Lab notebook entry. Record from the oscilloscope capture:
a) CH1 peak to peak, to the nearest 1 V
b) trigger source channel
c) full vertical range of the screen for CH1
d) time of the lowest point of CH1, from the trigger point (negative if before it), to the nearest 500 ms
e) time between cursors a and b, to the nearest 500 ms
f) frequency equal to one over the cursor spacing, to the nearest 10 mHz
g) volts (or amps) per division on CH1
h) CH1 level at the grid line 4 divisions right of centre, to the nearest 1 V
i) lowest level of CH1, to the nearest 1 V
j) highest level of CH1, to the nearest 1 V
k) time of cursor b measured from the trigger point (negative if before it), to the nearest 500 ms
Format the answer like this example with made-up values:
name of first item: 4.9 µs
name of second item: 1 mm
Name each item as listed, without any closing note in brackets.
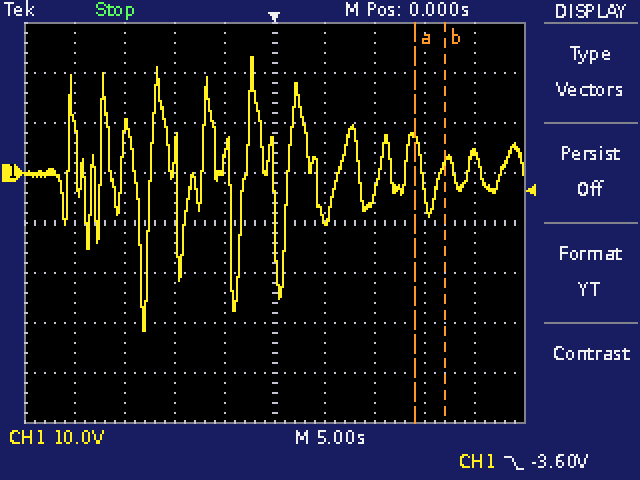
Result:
CH1 peak to peak, to the nearest 1 V: 55 V
trigger source channel: CH1
full vertical range of the screen for CH1: 80 V
time of the lowest point of CH1, from the trigger point (negative if before it), to the nearest 500 ms: -13.0 s
time between cursors a and b, to the nearest 500 ms: 3.0 s
frequency equal to one over the cursor spacing, to the nearest 10 mHz: 330 mHz
volts (or amps) per division on CH1: 10 V
CH1 level at the grid line 4 divisions right of centre, to the nearest 1 V: 4 V
lowest level of CH1, to the nearest 1 V: -32 V
highest level of CH1, to the nearest 1 V: 23 V
time of cursor b measured from the trigger point (negative if before it), to the nearest 500 ms: +17.0 s
